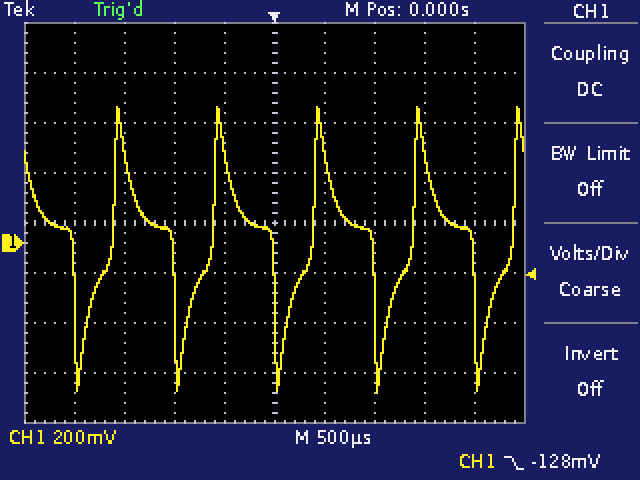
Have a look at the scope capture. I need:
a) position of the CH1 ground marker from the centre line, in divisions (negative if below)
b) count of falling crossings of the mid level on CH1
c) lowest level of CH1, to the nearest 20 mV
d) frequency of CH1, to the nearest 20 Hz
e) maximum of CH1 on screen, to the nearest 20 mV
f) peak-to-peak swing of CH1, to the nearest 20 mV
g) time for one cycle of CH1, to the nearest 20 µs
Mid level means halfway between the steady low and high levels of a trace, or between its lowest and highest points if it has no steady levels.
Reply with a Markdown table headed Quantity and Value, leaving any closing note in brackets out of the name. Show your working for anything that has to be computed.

| Quantity | Value |
|---|---|
| position of the CH1 ground marker from the centre line, in divisions | -0.4 div |
| count of falling crossings of the mid level on CH1 | 5 |
| lowest level of CH1, to the nearest 20 mV | -600 mV |
| frequency of CH1, to the nearest 20 Hz | 1 / 1.00 ms ≈ 1.00 kHz |
| maximum of CH1 on screen, to the nearest 20 mV | 540 mV |
| peak-to-peak swing of CH1, to the nearest 20 mV | 540 mV − (-600 mV) = 1.14 V |
| time for one cycle of CH1, to the nearest 20 µs | 1.00 ms |
